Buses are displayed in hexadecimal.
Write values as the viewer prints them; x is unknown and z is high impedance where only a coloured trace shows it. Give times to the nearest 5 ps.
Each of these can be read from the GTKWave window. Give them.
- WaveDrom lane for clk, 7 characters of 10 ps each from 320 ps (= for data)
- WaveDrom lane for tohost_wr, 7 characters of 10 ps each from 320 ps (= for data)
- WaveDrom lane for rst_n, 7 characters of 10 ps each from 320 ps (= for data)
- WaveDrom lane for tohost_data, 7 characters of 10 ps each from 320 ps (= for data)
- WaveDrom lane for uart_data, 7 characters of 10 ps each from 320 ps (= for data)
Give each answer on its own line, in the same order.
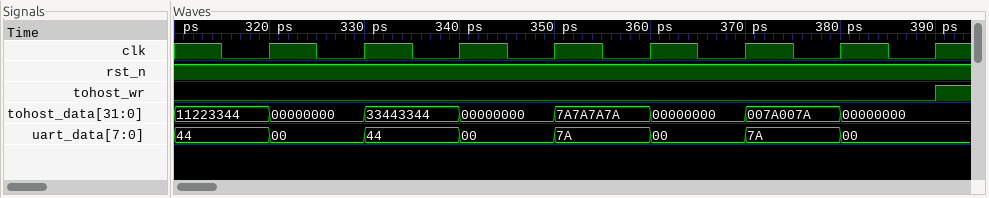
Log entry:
{name: 'clk', wave: 'p......'}
{name: 'tohost_wr', wave: '0......'}
{name: 'rst_n', wave: '1......'}
{name: 'tohost_data', wave: '=======', data: '00000000 33443344 00000000 7A7A7A7A 00000000 007A007A 00000000'}
{name: 'uart_data', wave: '=======', data: '00 44 00 7A 00 7A 00'}
